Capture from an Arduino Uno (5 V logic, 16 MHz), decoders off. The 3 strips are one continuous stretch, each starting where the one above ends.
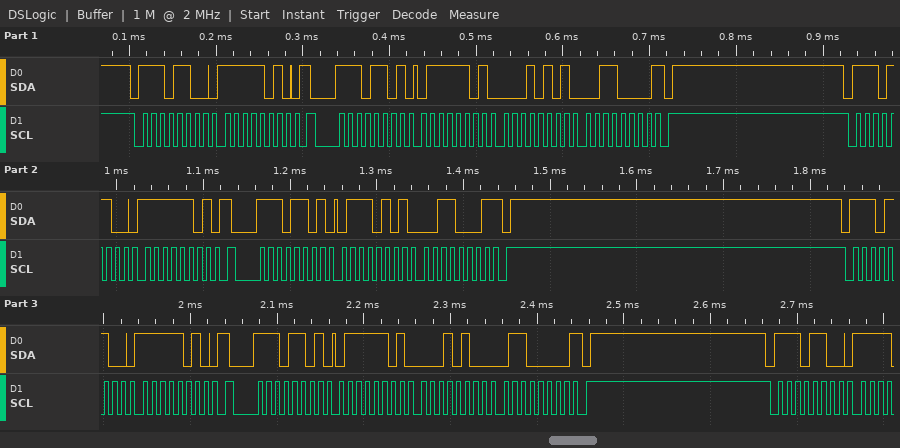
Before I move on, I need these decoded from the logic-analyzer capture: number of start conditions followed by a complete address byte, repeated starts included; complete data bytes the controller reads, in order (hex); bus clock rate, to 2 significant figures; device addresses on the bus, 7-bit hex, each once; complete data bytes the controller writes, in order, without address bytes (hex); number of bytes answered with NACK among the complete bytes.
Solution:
7
7D 15 30 75 31 7D 14 60
100 kHz
0x76
FA FD FA
3
